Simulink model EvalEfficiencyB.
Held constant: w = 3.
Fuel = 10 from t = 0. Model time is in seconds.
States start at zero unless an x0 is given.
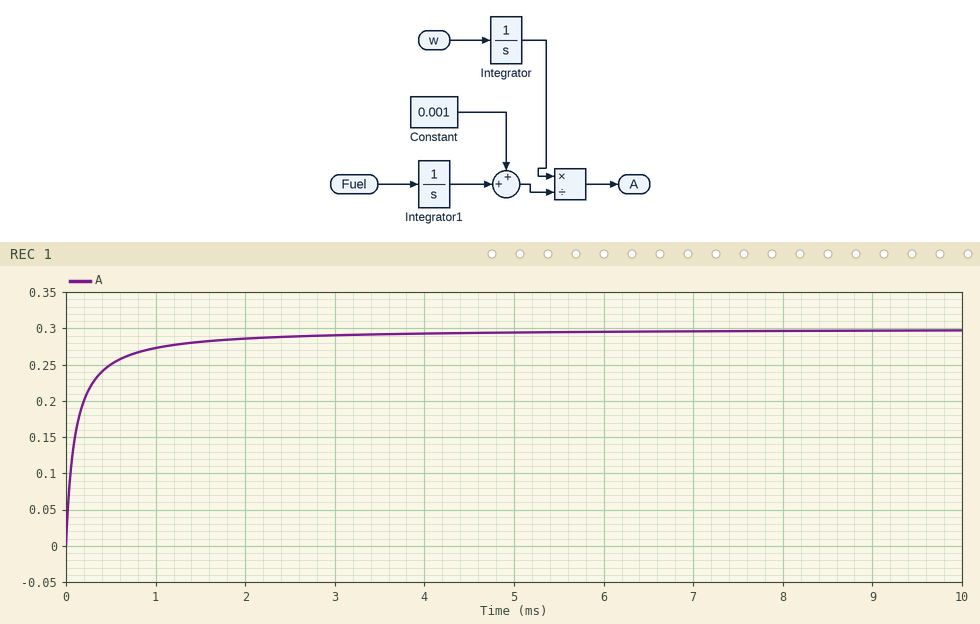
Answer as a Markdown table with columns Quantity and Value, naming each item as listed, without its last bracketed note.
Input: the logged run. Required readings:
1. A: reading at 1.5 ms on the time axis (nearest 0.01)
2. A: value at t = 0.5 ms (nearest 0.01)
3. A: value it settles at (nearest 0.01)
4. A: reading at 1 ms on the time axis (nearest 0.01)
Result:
| Quantity | Value |
|---|---|
| A: reading at 1.5 ms on the time axis | 0.28 |
| A: value at t = 0.5 ms | 0.25 |
| A: value it settles at | 0.30 |
| A: reading at 1 ms on the time axis | 0.27 |
